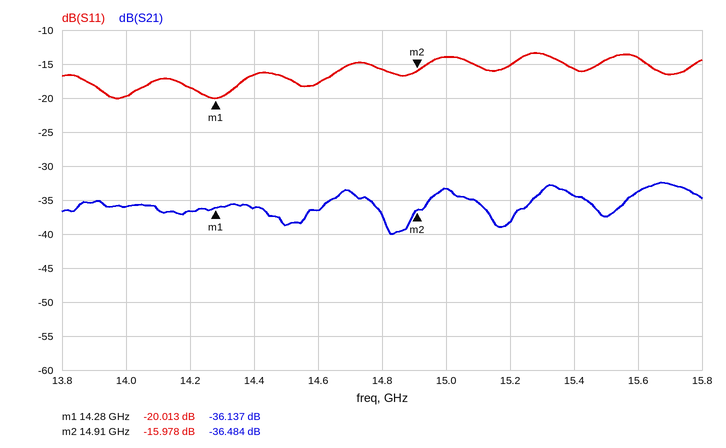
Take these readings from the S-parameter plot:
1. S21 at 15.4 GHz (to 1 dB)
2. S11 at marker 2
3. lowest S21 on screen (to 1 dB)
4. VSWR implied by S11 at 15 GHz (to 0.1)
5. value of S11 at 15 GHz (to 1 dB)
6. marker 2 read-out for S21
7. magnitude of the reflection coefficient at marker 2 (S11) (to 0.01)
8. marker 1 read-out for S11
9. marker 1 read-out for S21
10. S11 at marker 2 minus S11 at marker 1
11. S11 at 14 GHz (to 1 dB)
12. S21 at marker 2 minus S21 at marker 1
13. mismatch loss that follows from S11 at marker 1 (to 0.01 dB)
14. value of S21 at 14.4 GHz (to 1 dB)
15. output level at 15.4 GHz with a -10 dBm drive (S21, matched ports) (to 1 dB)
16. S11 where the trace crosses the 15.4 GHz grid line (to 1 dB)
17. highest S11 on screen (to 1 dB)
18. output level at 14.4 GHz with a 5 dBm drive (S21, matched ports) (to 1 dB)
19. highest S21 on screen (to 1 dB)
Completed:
-34 dB
-15.978 dB
-40 dB
1.5
-14 dB
-36.484 dB
0.16
-20.013 dB
-36.137 dB
4.035 dB
-20 dB
-0.347 dB
0.04 dB
-36 dB
-44 dBm
-16 dB
-13 dB
-31 dBm
-32 dB
